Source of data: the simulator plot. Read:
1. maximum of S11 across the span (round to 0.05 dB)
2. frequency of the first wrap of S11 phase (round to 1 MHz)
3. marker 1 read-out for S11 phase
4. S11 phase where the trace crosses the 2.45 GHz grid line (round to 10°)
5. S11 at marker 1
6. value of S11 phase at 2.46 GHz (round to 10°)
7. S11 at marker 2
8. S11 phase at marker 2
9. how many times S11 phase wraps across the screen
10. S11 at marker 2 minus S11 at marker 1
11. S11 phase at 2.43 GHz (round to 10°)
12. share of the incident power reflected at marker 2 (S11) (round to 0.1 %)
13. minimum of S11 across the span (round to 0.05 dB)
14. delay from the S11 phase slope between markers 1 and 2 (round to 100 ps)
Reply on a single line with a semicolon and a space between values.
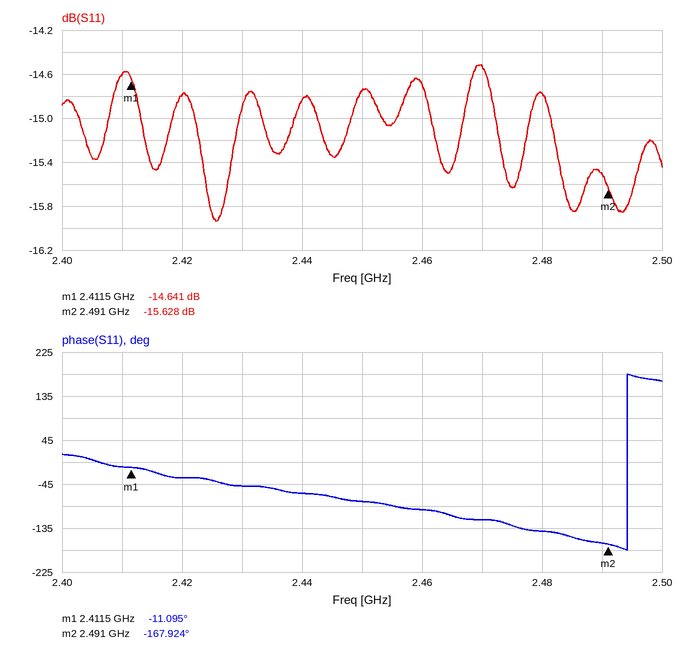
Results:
-14.50 dB; 2.494 GHz; -11.095°; -80°; -14.641 dB; -100°; -15.628 dB; -167.924°; 1; -0.987 dB; -50°; 2.7 %; -15.95 dB; 5.5 ns
